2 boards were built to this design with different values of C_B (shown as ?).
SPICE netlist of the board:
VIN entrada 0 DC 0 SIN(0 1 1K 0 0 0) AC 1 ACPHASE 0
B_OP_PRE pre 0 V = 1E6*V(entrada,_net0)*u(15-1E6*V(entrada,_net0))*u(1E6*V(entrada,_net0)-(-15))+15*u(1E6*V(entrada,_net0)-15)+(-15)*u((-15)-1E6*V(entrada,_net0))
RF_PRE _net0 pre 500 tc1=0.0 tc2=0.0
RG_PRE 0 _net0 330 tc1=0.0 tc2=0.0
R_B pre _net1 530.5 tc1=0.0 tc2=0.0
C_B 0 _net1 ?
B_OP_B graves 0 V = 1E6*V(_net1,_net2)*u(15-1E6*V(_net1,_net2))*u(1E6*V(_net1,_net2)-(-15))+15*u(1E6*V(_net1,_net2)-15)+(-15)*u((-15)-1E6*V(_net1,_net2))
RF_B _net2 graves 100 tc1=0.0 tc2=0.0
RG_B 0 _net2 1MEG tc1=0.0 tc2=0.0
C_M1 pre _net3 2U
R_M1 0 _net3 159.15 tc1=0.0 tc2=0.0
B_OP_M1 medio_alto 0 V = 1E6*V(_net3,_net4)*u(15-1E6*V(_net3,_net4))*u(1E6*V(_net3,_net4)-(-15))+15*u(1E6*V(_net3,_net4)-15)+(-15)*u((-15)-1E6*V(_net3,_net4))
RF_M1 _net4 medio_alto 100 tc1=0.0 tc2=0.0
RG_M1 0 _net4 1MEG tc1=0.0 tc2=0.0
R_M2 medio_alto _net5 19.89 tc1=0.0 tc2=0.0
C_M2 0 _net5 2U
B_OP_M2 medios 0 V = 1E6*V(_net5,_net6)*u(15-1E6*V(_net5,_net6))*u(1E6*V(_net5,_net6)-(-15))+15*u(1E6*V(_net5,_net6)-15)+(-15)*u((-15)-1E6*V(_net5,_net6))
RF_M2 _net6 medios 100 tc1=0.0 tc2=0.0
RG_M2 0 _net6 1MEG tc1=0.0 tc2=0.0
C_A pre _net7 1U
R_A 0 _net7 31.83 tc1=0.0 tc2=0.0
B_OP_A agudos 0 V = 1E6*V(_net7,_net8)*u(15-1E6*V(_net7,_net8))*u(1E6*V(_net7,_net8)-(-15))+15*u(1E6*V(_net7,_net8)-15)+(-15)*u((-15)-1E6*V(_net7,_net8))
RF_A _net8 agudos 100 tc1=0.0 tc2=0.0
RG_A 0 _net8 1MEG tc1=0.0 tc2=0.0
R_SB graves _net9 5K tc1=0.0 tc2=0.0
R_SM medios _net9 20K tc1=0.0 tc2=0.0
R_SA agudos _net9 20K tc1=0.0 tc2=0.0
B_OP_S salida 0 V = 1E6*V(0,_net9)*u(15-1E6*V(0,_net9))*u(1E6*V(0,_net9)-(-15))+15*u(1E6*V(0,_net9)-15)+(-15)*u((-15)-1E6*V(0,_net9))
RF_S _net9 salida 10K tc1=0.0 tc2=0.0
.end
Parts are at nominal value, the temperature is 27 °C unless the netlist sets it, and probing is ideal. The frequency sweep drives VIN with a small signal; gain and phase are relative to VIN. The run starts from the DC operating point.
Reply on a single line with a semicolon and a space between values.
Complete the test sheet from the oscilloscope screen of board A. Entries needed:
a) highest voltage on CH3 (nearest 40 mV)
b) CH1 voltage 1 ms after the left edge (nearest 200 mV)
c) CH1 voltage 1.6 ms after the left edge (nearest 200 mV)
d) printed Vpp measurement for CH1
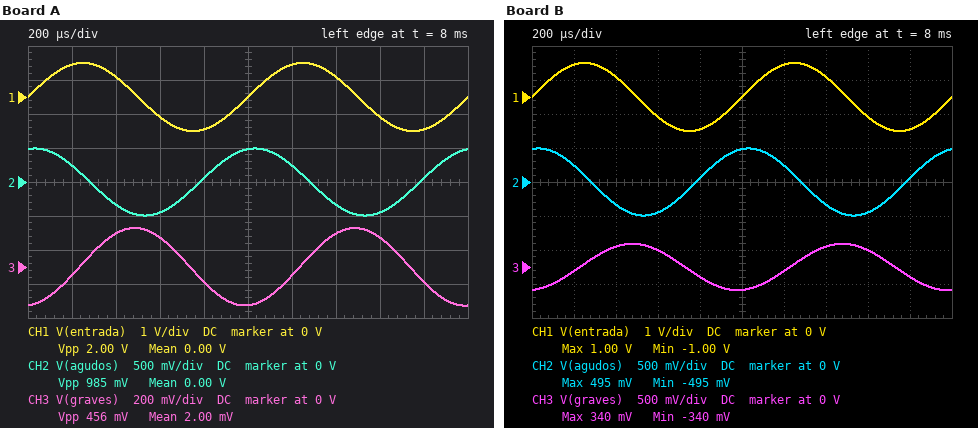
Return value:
240 mV; 0 V; -600 mV; 2.00 V
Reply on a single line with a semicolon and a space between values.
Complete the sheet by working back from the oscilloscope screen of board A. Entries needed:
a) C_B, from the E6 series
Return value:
3.3 µF
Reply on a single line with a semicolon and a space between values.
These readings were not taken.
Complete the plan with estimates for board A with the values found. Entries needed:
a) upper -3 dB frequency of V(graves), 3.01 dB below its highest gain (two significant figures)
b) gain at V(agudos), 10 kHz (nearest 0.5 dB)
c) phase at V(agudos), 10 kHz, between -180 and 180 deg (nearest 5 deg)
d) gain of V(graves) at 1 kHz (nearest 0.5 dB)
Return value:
91 Hz; 7.0 dB; 25 deg; -13.0 dB
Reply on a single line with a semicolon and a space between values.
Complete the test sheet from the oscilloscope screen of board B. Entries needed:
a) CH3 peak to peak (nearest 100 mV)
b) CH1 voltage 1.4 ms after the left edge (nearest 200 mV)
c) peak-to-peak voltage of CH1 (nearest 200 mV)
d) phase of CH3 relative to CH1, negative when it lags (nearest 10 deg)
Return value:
700 mV; 600 mV; 2.0 V; -80 deg
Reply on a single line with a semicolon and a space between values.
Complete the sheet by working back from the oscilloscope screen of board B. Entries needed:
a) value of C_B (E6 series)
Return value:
2.2 µF
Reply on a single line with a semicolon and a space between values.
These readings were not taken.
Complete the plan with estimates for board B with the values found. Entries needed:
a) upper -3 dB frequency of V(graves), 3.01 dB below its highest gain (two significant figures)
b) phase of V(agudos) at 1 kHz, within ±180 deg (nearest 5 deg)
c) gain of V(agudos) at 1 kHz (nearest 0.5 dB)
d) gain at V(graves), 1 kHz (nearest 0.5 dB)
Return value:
140 Hz; 80 deg; -6.0 dB; -9.5 dB
